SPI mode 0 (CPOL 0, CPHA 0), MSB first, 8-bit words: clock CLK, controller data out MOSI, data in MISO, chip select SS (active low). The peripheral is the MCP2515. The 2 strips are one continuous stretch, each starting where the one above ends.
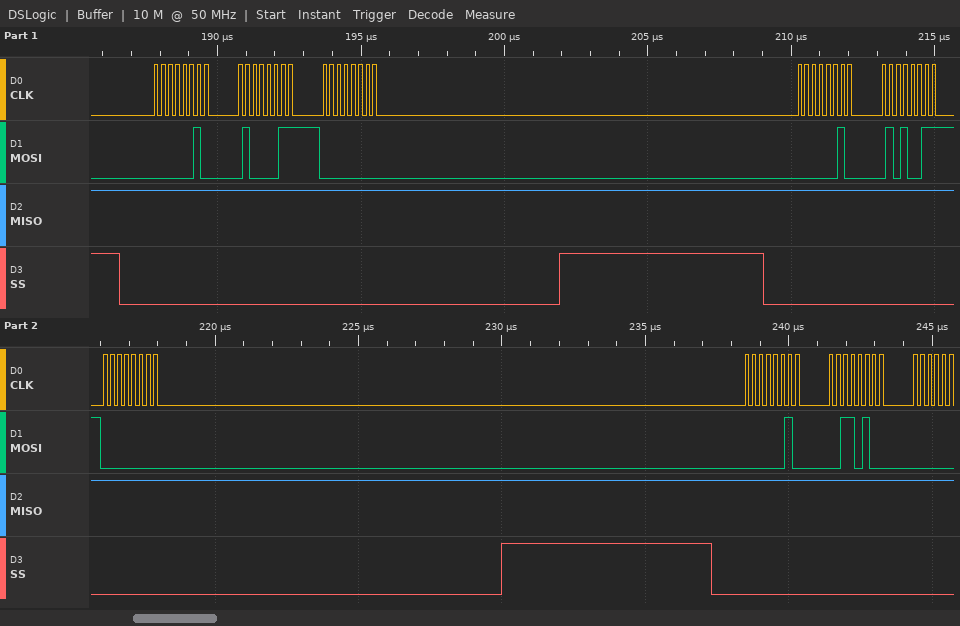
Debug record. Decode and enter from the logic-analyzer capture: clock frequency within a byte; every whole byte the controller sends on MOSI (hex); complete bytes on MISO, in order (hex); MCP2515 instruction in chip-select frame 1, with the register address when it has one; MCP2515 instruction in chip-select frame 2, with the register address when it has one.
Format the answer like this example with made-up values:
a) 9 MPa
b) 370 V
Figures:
a) 4 MHz
b) 02 43 00 02 53 00 02 34
c) FF FF FF FF FF FF FF FF
d) WRITE 0x43
e) WRITE 0x53
